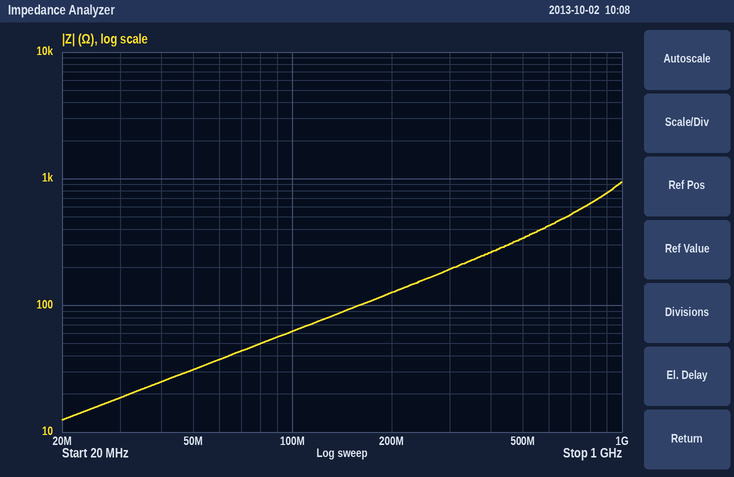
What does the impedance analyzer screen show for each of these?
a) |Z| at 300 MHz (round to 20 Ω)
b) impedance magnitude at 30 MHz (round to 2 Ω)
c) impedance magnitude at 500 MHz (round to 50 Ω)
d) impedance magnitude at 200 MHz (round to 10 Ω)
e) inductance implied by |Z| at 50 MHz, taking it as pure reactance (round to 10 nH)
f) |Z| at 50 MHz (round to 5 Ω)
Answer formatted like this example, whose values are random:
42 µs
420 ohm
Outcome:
200 Ω
18 Ω
350 Ω
130 Ω
100 nH
30 Ω
